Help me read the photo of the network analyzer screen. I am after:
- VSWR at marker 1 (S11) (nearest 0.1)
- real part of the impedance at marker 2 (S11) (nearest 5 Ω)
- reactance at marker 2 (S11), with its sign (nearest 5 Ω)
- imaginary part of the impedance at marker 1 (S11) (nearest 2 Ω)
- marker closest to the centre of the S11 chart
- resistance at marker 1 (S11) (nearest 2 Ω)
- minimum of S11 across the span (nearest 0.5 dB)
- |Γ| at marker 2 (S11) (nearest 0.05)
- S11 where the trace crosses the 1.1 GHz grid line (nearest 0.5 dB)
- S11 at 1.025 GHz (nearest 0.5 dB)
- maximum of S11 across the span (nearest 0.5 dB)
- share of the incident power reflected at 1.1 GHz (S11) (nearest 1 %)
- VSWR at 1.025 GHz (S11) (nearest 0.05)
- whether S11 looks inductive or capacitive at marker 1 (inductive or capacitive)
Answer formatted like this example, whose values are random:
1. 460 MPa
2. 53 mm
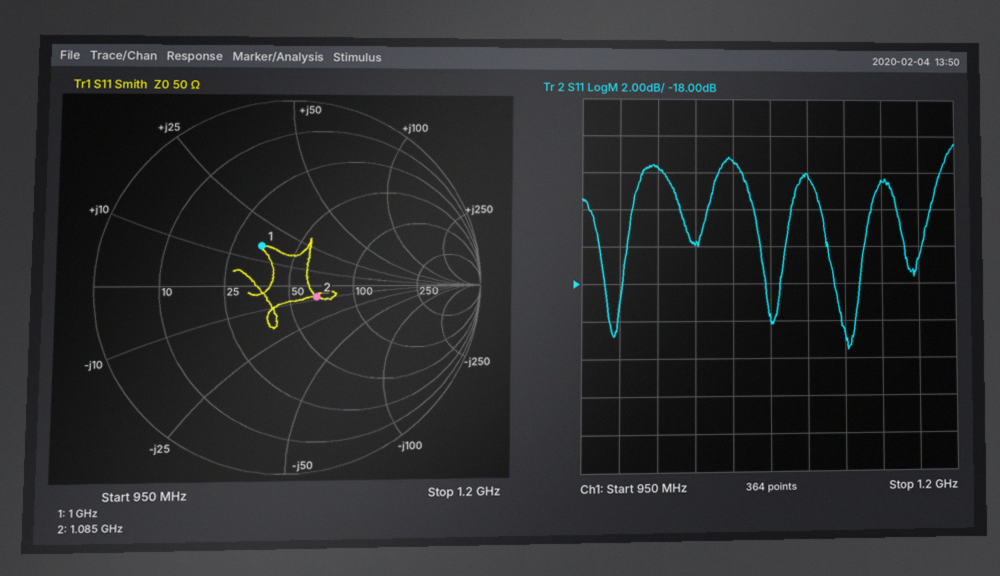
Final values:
1. 1.7
2. 65 Ω
3. -10 Ω
4. +16 Ω
5. marker 2
6. 34 Ω
7. -21.5 dB
8. 0.15
9. -12.0 dB
10. -16.0 dB
11. -10.5 dB
12. 6 %
13. 1.40
14. inductive
